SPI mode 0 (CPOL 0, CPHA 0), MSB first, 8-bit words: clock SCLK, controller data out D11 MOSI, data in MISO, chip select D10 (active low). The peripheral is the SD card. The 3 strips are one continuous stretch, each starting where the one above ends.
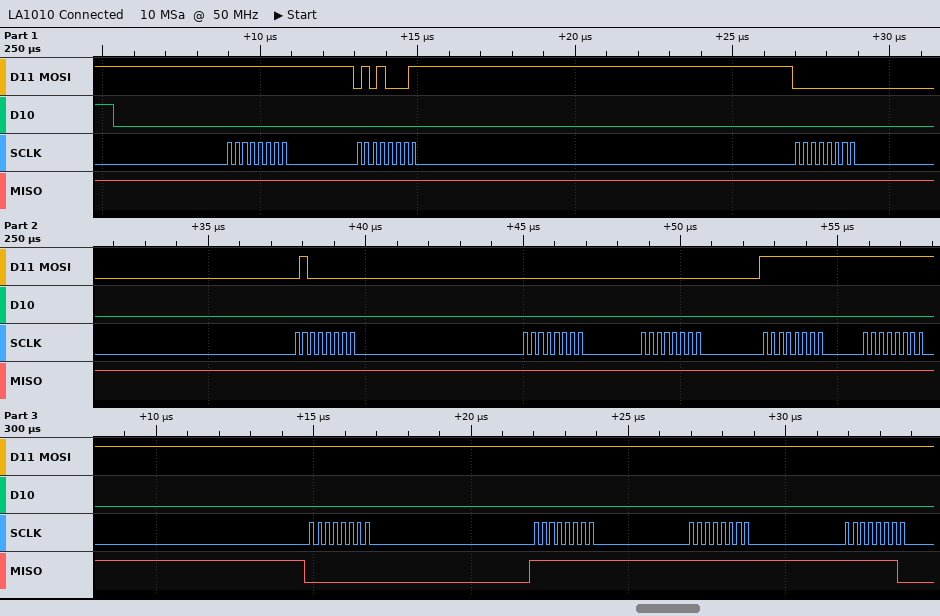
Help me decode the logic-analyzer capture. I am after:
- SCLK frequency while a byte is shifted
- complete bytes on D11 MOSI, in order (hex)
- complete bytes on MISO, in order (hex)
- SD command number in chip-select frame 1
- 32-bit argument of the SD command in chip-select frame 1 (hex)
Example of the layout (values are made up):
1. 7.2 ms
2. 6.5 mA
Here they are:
1. 4 MHz
2. 0xFF 0x51 0x00 0x40 0x00 0x00 0xFF 0xFF 0xFF 0xFF 0xFF 0xFF
3. 0xFF 0xFF 0xFF 0xFF 0xFF 0xFF 0xFF 0xFF 0x00 0xFF 0xFF 0xFE
4. CMD17
5. 0x00400000
